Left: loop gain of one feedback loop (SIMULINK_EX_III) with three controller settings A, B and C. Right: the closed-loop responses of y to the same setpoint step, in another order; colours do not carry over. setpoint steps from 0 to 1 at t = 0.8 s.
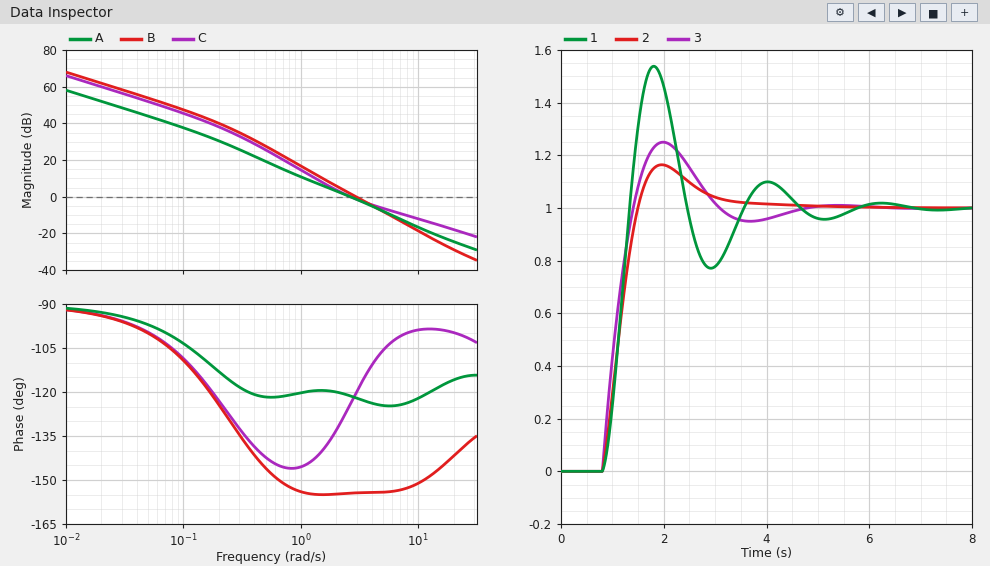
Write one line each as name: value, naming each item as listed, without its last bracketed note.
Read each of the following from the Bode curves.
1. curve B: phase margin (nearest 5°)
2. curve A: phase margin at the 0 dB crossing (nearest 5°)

curve B: phase margin: 25°
curve A: phase margin at the 0 dB crossing: 60°
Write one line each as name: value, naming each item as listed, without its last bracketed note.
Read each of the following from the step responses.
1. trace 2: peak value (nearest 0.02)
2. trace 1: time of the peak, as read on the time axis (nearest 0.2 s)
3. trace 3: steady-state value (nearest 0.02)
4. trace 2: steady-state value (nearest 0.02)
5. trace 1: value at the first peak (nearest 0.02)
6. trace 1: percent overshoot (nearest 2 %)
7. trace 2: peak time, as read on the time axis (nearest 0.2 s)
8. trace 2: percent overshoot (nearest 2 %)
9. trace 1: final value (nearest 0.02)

trace 2: peak value: 1.16
trace 1: time of the peak, as read on the time axis: 1.8 s
trace 3: steady-state value: 1.00
trace 2: steady-state value: 1.00
trace 1: value at the first peak: 1.54
trace 1: percent overshoot: 54 %
trace 2: peak time, as read on the time axis: 2.0 s
trace 2: percent overshoot: 16 %
trace 1: final value: 1.00
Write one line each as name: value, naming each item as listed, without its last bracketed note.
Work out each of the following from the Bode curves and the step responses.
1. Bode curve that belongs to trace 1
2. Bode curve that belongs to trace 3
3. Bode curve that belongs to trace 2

Bode curve that belongs to trace 1: B
Bode curve that belongs to trace 3: C
Bode curve that belongs to trace 2: A
